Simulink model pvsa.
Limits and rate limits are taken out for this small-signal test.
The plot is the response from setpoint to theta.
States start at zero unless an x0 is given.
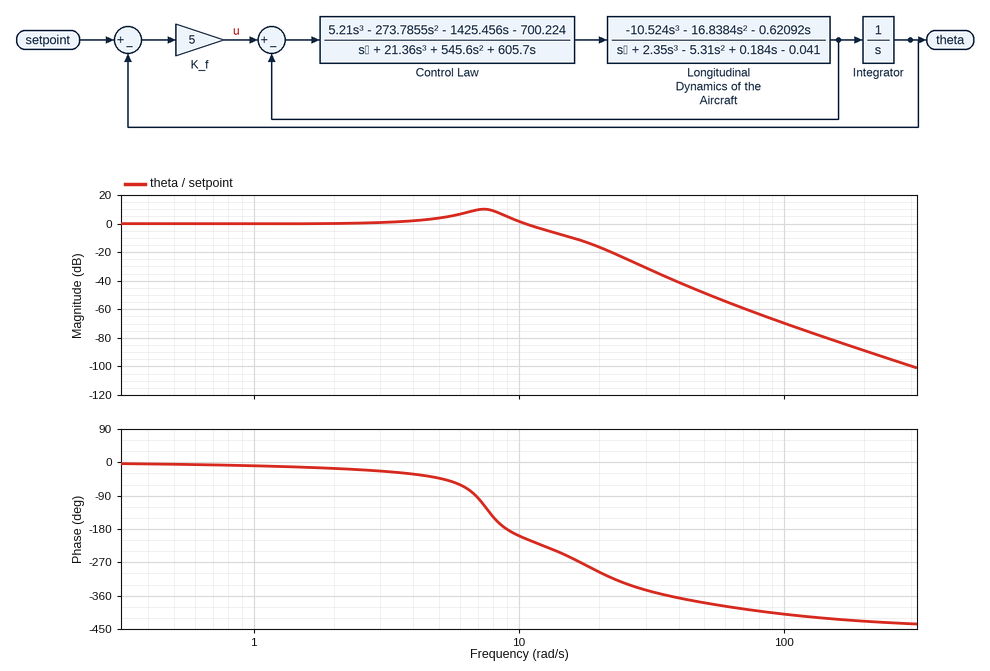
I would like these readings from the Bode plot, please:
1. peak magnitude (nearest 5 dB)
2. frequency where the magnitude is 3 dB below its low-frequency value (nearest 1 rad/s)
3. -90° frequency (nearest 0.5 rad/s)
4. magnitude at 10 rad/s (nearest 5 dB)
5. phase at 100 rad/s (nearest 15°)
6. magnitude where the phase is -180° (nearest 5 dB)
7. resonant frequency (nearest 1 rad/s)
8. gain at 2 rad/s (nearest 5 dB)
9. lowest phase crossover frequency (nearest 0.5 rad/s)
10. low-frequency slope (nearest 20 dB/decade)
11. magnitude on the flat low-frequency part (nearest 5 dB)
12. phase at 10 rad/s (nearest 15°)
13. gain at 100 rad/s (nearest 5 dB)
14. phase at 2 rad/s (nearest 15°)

10 dB
12 rad/s
7.0 rad/s
0 dB
-405°
5 dB
7 rad/s
0 dB
9.0 rad/s
0 dB/decade
0 dB
-195°
-70 dB
-15°
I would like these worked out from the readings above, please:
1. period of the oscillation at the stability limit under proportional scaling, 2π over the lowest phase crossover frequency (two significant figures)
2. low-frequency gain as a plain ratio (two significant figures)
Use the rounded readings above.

0.70 s
1.0
